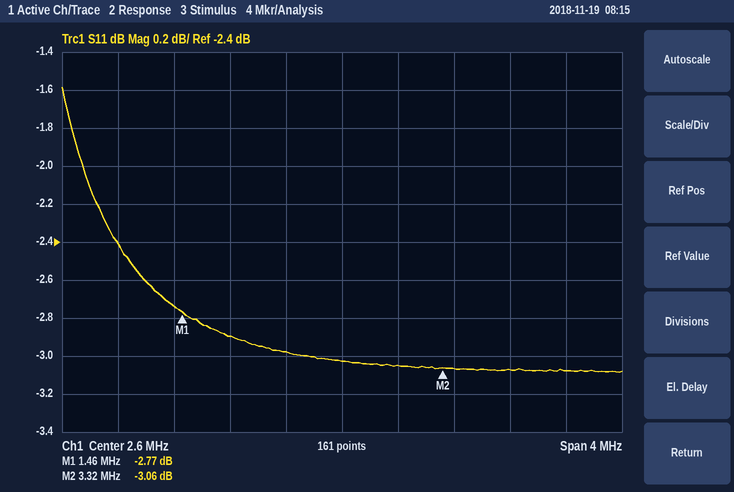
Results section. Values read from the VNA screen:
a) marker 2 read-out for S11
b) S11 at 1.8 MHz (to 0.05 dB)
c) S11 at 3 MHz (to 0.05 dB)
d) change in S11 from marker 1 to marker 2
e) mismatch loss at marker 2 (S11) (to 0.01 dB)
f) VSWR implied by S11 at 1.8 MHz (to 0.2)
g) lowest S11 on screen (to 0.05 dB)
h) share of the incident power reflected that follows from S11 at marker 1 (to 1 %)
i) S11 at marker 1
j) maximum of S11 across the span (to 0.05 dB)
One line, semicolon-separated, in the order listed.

-3.06 dB; -2.90 dB; -3.05 dB; -0.29 dB; 2.96 dB; 6.0; -3.10 dB; 53 %; -2.77 dB; -1.60 dB
